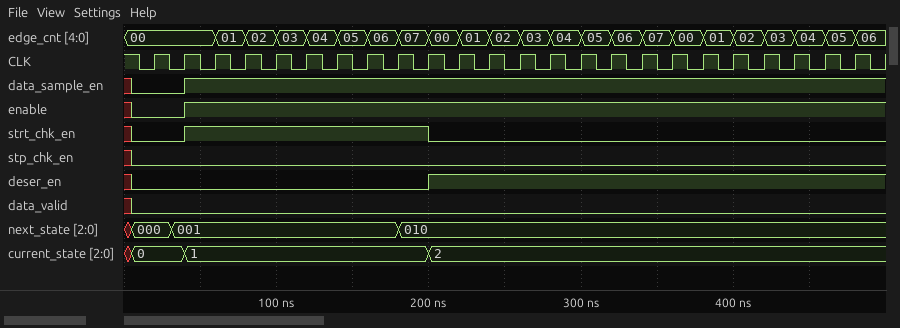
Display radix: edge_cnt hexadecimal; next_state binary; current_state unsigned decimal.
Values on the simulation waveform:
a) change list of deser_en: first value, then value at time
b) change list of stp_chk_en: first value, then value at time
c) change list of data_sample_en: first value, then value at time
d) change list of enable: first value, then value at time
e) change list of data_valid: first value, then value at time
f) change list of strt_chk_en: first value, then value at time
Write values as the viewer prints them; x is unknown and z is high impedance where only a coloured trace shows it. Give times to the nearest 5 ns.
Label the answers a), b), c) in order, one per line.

a) x, 0 at 5 ns, 1 at 200 ns
b) x, 0 at 5 ns
c) x, 0 at 5 ns, 1 at 40 ns
d) x, 0 at 5 ns, 1 at 40 ns
e) x, 0 at 5 ns
f) x, 0 at 5 ns, 1 at 40 ns, 0 at 200 ns
